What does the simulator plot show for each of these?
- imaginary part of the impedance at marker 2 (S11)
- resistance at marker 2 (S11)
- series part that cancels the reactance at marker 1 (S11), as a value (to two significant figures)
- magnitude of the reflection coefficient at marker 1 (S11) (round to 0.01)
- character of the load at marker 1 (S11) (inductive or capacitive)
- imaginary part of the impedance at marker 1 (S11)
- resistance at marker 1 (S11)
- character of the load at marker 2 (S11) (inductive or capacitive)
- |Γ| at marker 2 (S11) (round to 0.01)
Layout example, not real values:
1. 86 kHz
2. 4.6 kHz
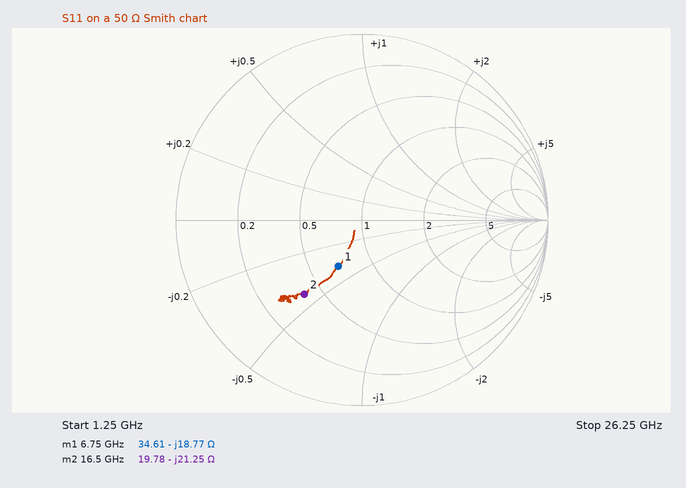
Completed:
1. -21.25 Ω
2. 19.78 Ω
3. 440 pH
4. 0.28
5. capacitive
6. -18.77 Ω
7. 34.61 Ω
8. capacitive
9. 0.51
